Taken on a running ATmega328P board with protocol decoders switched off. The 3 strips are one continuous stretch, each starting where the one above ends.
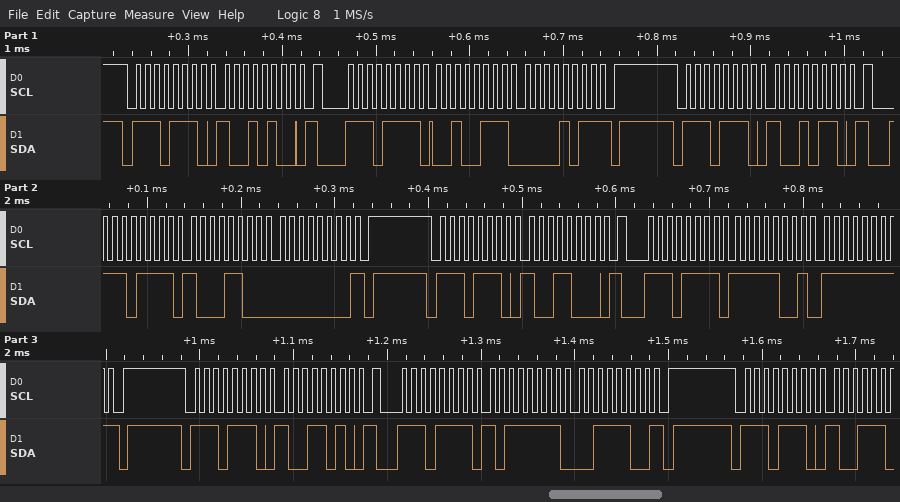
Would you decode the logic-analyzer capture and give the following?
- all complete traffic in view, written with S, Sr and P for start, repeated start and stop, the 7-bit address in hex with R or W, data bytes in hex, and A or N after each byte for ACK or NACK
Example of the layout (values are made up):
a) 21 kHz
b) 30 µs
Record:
a) S 77W A 94 A Sr 77R A 27 A 0B N P S 77W A 96 A Sr 77R A 8C A 00 N P S 77W A 98 A Sr 77R A F9 A FF N P S 77W A 9A A Sr 77R A BF A 3C N P S 77W A
